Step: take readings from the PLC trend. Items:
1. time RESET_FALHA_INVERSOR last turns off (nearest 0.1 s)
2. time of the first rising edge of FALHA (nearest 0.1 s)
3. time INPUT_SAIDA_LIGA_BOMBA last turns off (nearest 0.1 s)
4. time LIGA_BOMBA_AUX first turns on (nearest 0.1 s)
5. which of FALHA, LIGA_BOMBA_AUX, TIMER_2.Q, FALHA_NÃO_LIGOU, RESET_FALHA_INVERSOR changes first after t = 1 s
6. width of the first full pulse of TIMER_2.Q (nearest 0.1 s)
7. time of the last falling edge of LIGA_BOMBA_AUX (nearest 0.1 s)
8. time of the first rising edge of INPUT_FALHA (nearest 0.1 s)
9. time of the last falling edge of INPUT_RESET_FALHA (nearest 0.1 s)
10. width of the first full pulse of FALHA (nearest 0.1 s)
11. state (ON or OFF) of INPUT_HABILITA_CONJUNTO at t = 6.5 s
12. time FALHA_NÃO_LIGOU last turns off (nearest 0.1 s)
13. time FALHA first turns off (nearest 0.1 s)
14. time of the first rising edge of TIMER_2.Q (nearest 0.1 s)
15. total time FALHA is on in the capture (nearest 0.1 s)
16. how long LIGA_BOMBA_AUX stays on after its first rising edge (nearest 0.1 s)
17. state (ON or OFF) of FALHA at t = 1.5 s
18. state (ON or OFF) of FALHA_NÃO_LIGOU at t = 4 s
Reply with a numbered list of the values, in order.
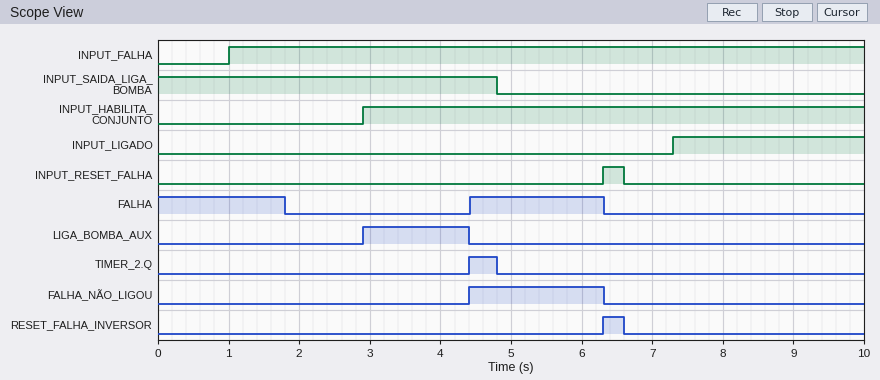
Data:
1. 6.6 s
2. 4.4 s
3. 4.8 s
4. 2.9 s
5. FALHA
6. 0.4 s
7. 4.4 s
8. 1.0 s
9. 6.6 s
10. 1.9 s
11. ON
12. 6.3 s
13. 1.8 s
14. 4.4 s
15. 3.7 s
16. 1.5 s
17. ON
18. OFF
